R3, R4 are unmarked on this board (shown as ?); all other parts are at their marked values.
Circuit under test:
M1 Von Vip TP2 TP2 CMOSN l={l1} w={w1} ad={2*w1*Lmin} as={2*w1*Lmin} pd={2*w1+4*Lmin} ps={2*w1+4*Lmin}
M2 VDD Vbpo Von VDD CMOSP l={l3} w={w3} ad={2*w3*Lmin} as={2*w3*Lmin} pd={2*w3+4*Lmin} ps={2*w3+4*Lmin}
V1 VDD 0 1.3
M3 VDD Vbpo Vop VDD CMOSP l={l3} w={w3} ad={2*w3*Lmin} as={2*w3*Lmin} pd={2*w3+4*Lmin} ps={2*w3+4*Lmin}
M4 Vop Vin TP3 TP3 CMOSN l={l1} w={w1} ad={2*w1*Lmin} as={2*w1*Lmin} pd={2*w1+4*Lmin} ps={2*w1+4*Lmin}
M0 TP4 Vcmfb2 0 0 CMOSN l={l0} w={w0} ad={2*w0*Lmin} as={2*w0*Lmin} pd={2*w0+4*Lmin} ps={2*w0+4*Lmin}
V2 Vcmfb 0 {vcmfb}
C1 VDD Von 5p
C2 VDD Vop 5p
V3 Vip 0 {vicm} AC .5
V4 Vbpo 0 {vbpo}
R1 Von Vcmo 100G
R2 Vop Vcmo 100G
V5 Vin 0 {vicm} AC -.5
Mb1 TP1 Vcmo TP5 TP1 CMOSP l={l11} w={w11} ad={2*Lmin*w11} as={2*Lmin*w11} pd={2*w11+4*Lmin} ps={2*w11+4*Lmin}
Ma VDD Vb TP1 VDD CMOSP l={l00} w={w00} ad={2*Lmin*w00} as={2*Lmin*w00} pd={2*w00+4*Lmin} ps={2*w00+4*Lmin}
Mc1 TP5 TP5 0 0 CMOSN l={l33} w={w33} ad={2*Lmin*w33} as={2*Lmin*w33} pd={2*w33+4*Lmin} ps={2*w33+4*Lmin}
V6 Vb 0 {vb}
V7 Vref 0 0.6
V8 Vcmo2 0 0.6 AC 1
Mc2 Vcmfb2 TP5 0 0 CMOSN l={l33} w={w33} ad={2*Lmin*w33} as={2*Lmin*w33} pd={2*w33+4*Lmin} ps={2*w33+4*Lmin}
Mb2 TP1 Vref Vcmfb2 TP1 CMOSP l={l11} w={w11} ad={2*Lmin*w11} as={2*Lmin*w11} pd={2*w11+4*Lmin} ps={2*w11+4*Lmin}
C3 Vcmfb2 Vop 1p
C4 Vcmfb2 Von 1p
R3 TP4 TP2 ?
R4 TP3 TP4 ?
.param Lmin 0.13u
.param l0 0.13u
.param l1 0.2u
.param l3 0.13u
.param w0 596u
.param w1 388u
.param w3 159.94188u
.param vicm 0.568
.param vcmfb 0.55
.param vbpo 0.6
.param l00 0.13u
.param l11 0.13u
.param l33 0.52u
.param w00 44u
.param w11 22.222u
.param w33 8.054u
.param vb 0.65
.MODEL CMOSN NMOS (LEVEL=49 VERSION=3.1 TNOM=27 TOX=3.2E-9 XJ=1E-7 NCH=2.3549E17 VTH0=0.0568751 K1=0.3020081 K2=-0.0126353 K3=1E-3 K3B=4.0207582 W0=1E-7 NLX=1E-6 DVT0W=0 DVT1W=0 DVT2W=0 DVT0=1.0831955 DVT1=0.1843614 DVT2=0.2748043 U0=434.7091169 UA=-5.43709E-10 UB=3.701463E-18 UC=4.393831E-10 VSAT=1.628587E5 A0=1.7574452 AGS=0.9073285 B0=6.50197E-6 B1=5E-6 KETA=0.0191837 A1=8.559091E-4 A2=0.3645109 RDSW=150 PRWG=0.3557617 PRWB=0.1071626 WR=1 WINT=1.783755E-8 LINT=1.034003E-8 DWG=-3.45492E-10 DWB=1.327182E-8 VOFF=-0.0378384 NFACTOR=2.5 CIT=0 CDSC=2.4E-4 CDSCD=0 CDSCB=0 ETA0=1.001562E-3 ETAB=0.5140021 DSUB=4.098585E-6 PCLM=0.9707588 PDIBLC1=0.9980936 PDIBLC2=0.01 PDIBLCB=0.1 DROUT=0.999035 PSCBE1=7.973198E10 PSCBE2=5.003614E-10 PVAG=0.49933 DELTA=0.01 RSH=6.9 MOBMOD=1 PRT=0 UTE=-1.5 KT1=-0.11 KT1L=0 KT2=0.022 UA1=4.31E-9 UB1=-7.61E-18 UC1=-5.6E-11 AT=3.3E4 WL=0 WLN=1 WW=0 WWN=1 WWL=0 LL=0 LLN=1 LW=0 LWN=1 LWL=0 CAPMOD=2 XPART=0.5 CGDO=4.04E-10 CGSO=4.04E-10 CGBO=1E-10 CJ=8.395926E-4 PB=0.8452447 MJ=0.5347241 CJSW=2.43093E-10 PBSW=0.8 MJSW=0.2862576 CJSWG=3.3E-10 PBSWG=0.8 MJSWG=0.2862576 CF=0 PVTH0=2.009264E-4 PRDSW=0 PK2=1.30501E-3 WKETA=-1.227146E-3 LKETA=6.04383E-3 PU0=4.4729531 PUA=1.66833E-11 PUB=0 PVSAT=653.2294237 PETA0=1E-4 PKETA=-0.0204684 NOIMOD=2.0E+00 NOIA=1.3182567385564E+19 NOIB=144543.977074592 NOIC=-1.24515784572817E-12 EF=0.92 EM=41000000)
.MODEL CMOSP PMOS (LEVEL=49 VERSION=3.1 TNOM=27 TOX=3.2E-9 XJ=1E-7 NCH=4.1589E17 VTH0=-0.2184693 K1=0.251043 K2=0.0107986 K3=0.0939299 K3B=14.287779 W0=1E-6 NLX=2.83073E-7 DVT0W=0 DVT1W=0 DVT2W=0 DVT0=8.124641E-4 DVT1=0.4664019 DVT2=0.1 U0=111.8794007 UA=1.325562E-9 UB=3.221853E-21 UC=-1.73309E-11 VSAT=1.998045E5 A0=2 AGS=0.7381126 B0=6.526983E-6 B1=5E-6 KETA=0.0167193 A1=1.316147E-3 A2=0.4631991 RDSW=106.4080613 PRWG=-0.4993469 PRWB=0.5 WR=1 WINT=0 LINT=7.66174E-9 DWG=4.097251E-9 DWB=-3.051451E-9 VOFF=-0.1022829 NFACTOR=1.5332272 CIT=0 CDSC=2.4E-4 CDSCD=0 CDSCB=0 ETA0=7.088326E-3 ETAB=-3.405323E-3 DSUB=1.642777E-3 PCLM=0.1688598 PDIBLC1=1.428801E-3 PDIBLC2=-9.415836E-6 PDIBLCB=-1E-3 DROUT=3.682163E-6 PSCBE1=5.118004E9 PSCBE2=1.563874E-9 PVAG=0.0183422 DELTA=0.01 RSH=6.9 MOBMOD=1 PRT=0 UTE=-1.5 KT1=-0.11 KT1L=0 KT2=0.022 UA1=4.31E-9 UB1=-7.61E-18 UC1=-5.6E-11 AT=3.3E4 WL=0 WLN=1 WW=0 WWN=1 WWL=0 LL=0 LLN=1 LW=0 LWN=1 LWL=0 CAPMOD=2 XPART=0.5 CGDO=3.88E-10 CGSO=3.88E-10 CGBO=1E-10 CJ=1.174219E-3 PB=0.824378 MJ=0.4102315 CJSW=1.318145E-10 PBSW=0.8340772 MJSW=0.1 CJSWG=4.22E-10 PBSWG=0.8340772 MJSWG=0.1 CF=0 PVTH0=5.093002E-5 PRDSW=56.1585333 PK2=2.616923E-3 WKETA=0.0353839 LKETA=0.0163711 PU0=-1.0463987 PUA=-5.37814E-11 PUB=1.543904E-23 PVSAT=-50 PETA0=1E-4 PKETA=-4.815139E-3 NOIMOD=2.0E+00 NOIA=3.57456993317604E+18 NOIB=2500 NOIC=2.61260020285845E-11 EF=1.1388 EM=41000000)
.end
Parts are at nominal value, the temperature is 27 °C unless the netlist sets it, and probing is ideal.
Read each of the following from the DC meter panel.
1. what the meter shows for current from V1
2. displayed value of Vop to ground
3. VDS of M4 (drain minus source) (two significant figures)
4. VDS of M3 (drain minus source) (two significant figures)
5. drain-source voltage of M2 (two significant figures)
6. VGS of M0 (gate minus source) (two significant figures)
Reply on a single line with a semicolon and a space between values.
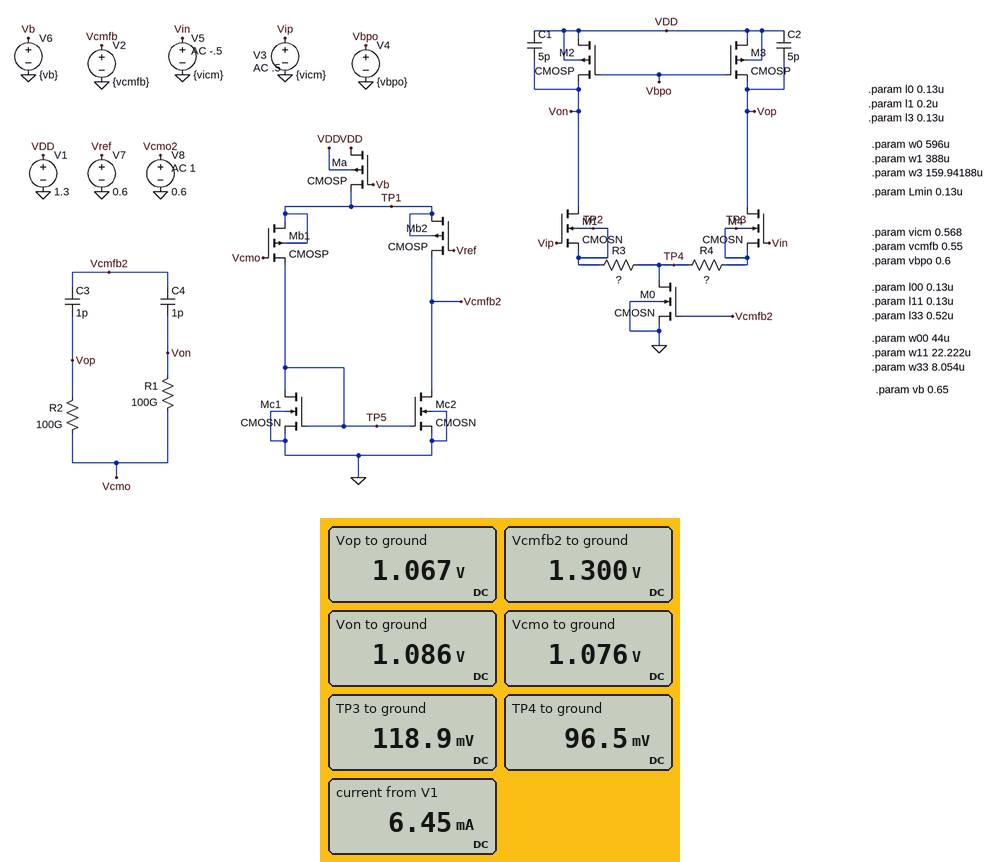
6.45 mA; 1.067 V; 950 mV; 230 mV; 210 mV; 1.3 V
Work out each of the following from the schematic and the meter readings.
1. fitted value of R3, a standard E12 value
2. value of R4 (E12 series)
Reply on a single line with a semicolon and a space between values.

8.2 Ω; 6.8 Ω
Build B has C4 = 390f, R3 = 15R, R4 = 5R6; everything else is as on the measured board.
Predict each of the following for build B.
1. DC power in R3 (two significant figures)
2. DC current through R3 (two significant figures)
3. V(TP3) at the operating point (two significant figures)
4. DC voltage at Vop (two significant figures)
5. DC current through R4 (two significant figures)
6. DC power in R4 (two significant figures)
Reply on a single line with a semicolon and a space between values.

110 µW; 2.7 mA; 110 mV; 1.0 V; 3.5 mA; 69 µW
